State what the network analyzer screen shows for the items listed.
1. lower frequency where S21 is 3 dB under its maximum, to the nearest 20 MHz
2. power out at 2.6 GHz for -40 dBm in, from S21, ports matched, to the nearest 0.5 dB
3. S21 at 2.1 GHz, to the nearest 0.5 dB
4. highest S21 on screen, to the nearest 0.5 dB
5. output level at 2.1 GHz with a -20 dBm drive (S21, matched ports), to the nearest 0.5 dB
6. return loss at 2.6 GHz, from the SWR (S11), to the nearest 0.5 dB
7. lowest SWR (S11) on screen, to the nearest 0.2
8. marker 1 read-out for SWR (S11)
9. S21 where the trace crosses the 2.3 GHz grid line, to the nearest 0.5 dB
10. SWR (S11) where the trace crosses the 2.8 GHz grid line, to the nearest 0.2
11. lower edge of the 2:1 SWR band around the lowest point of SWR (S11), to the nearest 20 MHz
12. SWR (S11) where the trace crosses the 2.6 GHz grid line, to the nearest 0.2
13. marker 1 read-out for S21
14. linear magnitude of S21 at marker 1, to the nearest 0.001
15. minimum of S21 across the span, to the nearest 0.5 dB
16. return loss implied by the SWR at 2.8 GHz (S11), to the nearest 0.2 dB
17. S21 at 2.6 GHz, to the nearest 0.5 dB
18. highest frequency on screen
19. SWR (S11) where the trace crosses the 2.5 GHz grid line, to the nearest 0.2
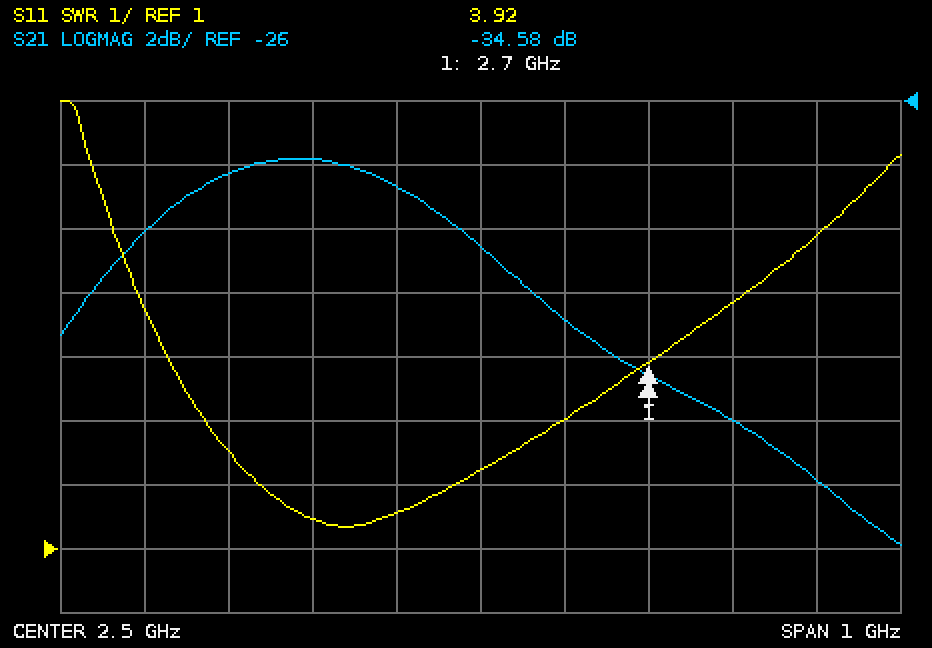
2.08 GHz
-73.0 dBm
-30.0 dB
-28.0 dB
-50.0 dBm
6.0 dB
1.4
3.92
-28.0 dB
4.8
2.24 GHz
3.0
-34.58 dB
0.019
-40.0 dB
3.6 dB
-33.0 dB
3 GHz
2.2
